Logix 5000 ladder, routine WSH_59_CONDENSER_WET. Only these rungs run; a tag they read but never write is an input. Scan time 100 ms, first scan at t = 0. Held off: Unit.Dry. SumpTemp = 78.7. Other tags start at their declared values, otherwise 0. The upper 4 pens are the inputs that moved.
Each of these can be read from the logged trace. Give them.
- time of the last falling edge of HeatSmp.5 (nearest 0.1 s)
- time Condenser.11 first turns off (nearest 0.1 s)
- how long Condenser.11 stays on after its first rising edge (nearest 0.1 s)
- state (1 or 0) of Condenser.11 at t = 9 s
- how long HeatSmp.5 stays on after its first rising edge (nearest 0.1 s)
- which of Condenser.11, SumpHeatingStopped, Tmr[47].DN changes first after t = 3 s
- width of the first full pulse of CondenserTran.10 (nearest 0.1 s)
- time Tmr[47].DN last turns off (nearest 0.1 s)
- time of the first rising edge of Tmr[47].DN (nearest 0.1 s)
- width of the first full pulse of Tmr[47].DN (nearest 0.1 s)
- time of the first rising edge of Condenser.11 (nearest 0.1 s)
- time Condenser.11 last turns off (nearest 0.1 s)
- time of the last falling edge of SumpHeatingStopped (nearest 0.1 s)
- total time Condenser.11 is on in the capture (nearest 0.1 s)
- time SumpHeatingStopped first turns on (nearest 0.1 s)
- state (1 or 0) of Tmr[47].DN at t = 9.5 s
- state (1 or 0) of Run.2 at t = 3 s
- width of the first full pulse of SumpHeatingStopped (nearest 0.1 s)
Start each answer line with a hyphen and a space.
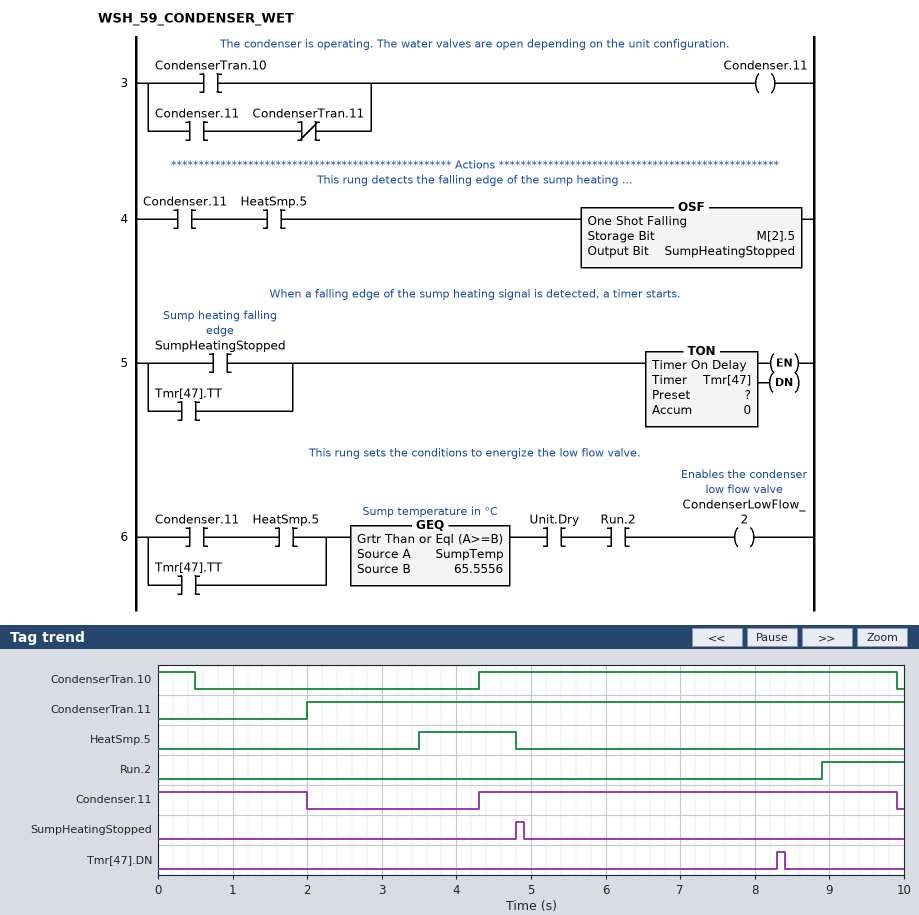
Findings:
- 4.8 s
- 2.0 s
- 5.6 s
- 1
- 1.3 s
- Condenser.11
- 5.6 s
- 8.4 s
- 8.3 s
- 0.1 s
- 4.3 s
- 9.9 s
- 4.9 s
- 7.6 s
- 4.8 s
- 0
- 0
- 0.1 s
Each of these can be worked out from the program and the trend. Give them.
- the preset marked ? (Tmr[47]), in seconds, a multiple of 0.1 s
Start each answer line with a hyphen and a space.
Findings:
- 3.5 s
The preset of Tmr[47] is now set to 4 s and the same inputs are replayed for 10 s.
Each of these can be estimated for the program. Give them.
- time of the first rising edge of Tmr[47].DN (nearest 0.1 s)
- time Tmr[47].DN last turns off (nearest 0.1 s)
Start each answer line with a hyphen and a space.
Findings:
- 8.8 s
- 8.9 s
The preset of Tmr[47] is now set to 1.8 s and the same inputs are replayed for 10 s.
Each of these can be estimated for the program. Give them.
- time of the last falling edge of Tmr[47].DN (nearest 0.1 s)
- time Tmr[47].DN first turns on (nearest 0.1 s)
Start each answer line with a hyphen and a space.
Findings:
- 6.7 s
- 6.6 s
